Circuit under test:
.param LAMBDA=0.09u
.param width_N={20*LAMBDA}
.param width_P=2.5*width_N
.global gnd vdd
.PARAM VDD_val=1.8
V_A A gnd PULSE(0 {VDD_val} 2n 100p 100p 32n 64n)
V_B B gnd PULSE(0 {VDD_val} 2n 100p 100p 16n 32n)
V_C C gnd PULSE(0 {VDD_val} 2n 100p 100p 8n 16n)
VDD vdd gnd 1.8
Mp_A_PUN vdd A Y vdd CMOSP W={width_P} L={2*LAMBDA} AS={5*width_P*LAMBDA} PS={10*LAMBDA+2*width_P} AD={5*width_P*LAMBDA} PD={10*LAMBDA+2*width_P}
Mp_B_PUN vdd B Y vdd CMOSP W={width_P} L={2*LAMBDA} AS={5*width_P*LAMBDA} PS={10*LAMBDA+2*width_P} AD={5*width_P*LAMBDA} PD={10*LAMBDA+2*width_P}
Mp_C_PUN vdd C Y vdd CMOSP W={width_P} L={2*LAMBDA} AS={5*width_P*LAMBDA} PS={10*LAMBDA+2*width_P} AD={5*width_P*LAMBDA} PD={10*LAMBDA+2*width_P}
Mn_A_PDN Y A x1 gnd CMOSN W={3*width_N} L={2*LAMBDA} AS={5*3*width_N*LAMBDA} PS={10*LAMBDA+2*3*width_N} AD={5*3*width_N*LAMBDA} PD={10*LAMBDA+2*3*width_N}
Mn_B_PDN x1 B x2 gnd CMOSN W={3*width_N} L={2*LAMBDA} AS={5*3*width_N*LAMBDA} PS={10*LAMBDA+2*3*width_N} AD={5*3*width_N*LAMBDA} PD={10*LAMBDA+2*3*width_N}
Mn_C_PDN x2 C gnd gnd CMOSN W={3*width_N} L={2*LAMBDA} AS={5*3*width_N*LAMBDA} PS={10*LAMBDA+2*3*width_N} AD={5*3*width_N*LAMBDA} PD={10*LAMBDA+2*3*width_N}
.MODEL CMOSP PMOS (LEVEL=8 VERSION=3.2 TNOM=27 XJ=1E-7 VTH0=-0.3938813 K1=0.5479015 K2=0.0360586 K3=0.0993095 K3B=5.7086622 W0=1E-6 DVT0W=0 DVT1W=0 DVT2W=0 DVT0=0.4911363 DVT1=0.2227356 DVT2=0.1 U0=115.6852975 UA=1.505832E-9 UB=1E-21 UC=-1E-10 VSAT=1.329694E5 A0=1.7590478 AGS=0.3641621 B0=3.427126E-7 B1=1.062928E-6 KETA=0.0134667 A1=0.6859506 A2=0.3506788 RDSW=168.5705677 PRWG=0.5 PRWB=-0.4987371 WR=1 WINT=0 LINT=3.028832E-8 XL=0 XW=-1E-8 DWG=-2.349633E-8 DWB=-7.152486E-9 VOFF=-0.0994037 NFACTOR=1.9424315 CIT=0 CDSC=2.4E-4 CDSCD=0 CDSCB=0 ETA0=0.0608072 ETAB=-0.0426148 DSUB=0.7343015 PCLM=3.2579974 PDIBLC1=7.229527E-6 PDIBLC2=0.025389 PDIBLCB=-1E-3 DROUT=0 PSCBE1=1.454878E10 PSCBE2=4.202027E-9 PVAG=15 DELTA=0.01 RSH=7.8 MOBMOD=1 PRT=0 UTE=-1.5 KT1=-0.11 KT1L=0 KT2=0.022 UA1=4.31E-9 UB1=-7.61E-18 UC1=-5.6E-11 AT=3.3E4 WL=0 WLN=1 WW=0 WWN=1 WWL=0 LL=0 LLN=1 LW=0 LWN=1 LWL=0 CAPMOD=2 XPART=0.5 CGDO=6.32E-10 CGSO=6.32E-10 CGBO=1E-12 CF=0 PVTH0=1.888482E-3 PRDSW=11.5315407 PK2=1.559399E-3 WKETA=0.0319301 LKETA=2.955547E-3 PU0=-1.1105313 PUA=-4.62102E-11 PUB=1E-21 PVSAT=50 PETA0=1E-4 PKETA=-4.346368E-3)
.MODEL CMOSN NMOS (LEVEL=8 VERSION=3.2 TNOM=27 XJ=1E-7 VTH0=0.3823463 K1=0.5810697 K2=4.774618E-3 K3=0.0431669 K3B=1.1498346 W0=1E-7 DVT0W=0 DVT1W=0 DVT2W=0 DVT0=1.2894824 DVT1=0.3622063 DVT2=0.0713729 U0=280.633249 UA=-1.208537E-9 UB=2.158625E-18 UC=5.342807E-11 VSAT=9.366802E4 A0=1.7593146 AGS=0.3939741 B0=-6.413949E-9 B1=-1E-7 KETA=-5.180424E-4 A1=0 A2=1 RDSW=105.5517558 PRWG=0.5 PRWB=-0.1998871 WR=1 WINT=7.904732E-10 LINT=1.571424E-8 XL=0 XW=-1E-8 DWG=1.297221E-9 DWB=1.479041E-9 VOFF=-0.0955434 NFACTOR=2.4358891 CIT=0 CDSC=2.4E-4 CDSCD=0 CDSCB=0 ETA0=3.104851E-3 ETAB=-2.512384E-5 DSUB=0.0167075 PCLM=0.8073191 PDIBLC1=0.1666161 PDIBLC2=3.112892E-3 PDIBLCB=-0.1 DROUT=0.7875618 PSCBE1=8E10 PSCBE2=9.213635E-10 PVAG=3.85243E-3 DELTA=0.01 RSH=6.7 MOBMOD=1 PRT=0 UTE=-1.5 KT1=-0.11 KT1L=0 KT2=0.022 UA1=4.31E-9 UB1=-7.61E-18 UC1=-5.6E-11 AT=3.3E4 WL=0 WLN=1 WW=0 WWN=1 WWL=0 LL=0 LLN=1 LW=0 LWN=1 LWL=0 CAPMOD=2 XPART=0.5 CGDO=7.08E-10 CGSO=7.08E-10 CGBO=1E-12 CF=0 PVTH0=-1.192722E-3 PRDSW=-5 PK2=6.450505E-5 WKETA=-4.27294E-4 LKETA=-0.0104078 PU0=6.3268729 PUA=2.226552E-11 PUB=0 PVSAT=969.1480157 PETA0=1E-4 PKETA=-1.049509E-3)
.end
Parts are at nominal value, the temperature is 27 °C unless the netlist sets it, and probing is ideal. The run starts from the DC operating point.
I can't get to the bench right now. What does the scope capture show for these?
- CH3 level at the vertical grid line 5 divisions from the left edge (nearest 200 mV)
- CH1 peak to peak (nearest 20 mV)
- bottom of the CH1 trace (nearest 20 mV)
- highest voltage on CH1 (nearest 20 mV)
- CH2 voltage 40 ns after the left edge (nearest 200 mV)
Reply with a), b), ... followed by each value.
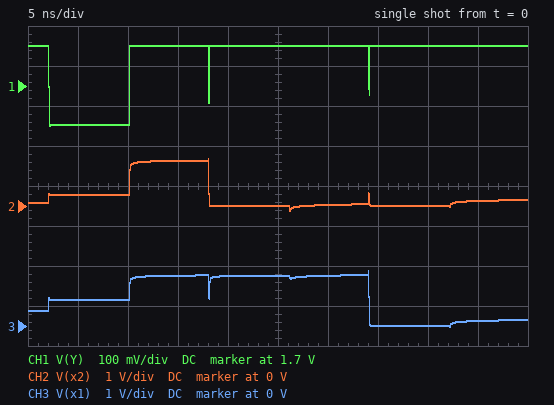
a) 1.2 V
b) 200 mV
c) 1.60 V
d) 1.80 V
e) 0 V
